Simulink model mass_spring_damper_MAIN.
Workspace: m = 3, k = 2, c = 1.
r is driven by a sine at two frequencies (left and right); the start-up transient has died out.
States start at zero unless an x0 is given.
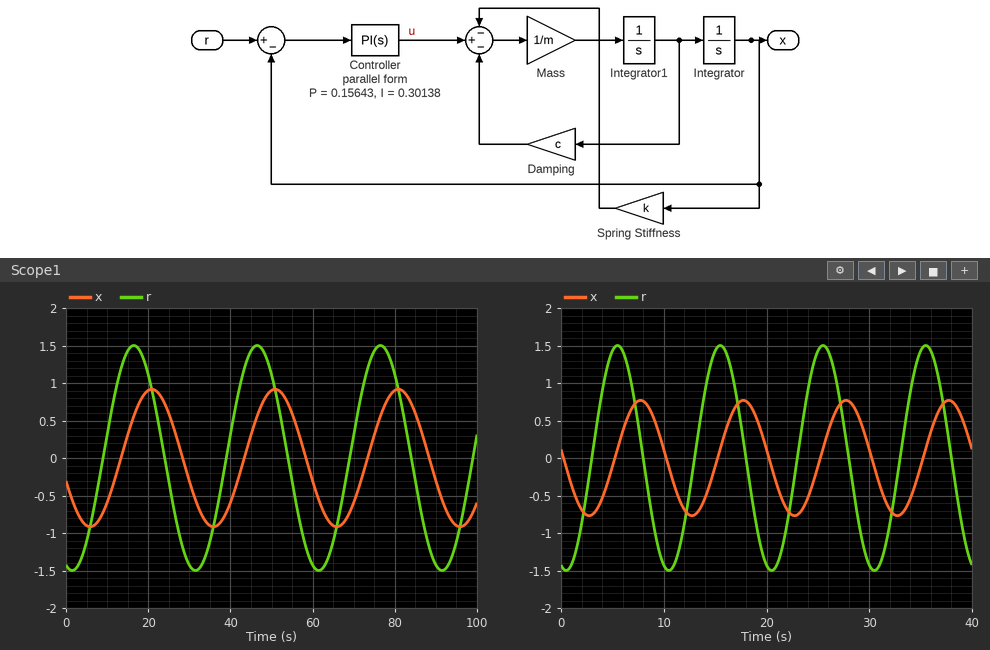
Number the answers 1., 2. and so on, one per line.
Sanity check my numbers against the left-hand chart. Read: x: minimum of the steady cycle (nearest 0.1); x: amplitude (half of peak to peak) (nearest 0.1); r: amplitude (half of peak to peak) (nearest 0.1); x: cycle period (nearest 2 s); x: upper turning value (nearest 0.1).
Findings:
1. -0.9
2. 0.9
3. 1.5
4. 30 s
5. 0.9
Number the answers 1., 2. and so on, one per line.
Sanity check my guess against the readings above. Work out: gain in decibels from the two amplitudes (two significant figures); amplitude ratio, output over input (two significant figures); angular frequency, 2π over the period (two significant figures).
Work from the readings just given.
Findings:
1. -4.4 dB
2. 0.60
3. 0.21 rad/s
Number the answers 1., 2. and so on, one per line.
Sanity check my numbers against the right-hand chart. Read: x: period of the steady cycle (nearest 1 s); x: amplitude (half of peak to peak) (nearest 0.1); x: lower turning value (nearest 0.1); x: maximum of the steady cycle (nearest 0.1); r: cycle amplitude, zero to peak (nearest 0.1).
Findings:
1. 10 s
2. 0.8
3. -0.8
4. 0.8
5. 1.5
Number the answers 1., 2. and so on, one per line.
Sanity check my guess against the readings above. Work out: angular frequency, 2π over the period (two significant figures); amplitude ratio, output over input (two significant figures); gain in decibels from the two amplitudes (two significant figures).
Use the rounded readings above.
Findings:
1. 0.63 rad/s
2. 0.53
3. -5.5 dB
